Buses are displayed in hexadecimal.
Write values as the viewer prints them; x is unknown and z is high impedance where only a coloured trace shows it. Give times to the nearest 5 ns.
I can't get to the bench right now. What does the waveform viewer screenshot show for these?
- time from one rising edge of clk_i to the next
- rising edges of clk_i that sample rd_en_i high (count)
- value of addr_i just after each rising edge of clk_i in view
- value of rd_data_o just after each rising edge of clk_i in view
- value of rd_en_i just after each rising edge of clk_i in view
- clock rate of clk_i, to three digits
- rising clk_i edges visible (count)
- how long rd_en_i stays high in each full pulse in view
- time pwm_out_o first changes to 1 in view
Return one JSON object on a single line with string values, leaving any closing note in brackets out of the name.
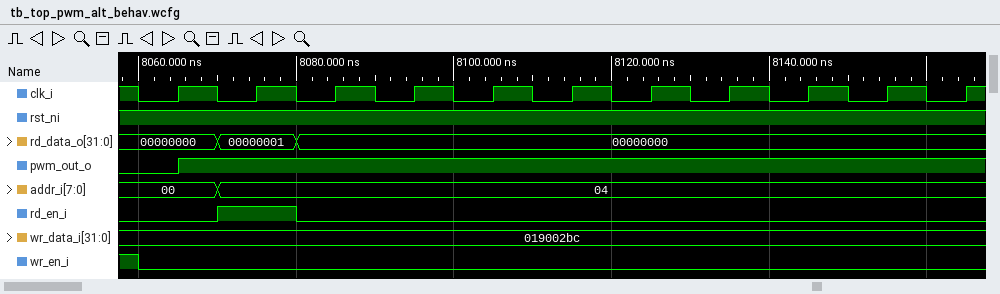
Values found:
{"time from one rising edge of clk_i to the next": "10 ns", "rising edges of clk_i that sample rd_en_i high": "1", "value of addr_i just after each rising edge of clk_i in view": "00, 04, 04, 04, 04, 04, 04, 04, 04, 04, 04", "value of rd_data_o just after each rising edge of clk_i in view": "00000000, 00000001, 00000000, 00000000, 00000000, 00000000, 00000000, 00000000, 00000000, 00000000, 00000000", "value of rd_en_i just after each rising edge of clk_i in view": "0 1 0 0 0 0 0 0 0 0 0", "clock rate of clk_i, to three digits": "100 MHz", "rising clk_i edges visible": "11", "how long rd_en_i stays high in each full pulse in view": "10 ns", "time pwm_out_o first changes to 1 in view": "8065 ns"}
